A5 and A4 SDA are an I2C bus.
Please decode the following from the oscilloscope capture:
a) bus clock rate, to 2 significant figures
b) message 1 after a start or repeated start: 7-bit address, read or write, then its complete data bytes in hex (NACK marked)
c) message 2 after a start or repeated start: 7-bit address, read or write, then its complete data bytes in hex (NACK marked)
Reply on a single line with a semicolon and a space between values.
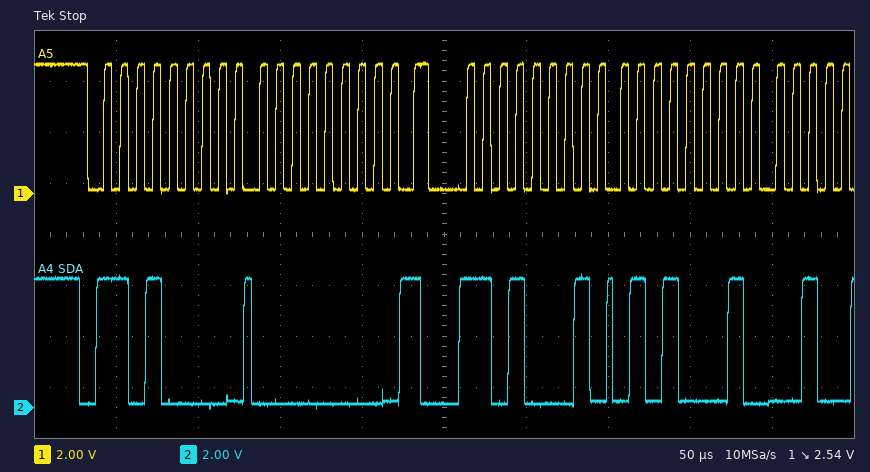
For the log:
100 kHz; 0x68 write: 00; 0x68 read: 51
